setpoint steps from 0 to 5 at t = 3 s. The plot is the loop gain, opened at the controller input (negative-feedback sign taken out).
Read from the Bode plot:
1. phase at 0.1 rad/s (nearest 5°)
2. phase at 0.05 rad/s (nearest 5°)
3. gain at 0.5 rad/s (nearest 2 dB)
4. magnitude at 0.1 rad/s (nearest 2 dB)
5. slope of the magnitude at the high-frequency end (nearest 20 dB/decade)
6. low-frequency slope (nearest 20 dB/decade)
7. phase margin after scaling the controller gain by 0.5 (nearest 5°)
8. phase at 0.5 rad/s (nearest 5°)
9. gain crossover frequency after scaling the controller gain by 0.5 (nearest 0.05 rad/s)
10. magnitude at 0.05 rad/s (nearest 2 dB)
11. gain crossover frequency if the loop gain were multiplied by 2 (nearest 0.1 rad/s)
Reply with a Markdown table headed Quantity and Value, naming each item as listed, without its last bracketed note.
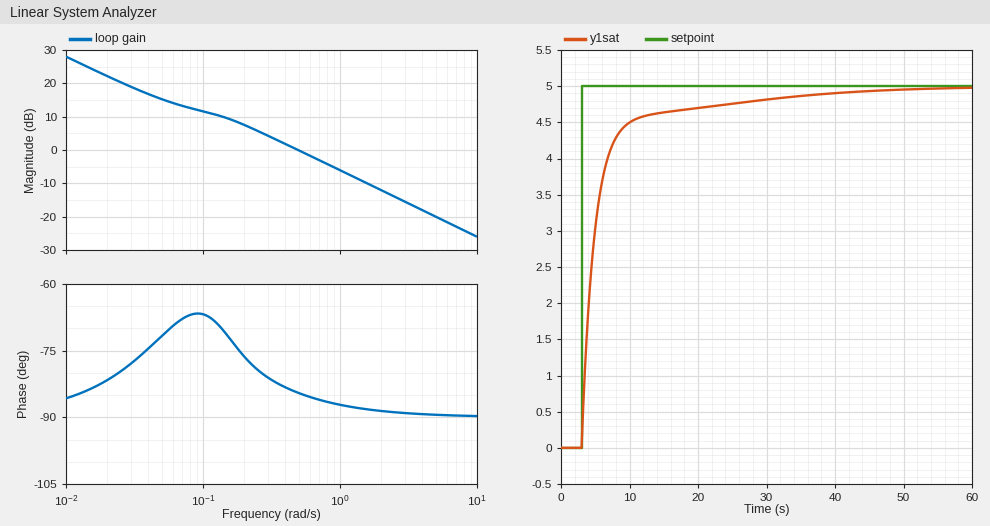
| Quantity | Value |
|---|---|
| phase at 0.1 rad/s | -65° |
| phase at 0.05 rad/s | -70° |
| gain at 0.5 rad/s | 0 dB |
| magnitude at 0.1 rad/s | 12 dB |
| slope of the magnitude at the high-frequency end | -20 dB/decade |
| low-frequency slope | -20 dB/decade |
| phase margin after scaling the controller gain by 0.5 | 100° |
| phase at 0.5 rad/s | -85° |
| gain crossover frequency after scaling the controller gain by 0.5 | 0.25 rad/s |
| magnitude at 0.05 rad/s | 16 dB |
| gain crossover frequency if the loop gain were multiplied by 2 | 1.0 rad/s |
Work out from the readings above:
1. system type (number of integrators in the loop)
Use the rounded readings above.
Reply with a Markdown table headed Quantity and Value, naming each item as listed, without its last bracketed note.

| Quantity | Value |
|---|---|
| system type | 1 |
